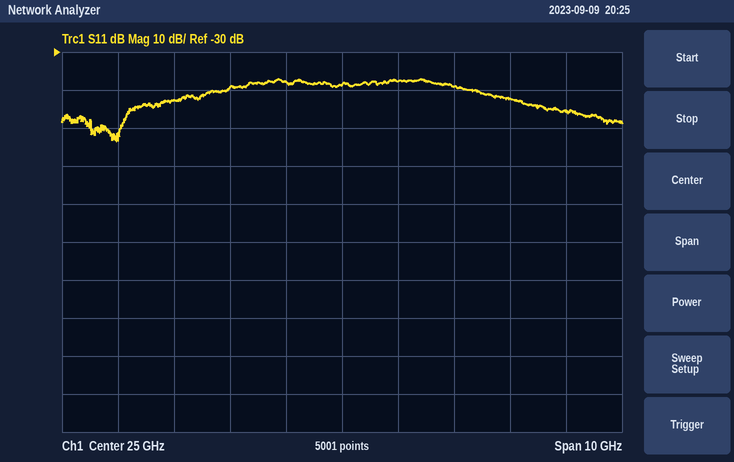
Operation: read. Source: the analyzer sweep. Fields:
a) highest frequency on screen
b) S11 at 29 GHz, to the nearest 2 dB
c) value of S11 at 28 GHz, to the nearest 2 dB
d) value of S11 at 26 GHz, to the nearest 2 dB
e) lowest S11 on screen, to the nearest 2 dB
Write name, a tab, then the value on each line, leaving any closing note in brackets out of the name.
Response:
highest frequency on screen	30 GHz
S11 at 29 GHz, to the nearest 2 dB	-46 dB
value of S11 at 28 GHz, to the nearest 2 dB	-42 dB
value of S11 at 26 GHz, to the nearest 2 dB	-38 dB
lowest S11 on screen, to the nearest 2 dB	-54 dB
